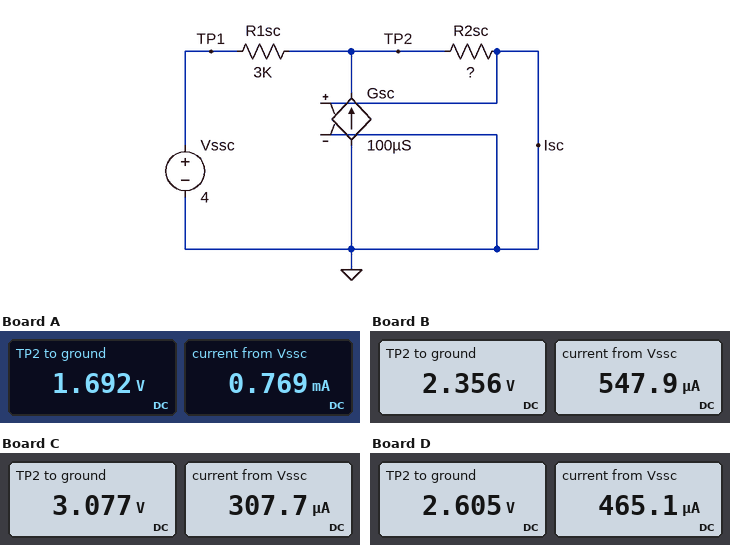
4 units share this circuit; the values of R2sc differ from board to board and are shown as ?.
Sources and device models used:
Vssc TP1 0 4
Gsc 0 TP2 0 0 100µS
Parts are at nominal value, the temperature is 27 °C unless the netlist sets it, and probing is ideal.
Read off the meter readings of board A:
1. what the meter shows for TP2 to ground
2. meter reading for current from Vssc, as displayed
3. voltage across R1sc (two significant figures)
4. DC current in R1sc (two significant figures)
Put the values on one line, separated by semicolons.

1.692 V; 0.769 mA; 2.3 V; 770 µA
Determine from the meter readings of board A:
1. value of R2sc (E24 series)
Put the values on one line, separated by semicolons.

2.2 kΩ
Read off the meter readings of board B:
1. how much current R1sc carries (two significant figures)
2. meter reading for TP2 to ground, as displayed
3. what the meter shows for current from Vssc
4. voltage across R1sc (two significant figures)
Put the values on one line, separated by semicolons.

550 µA; 2.356 V; 547.9 µA; 1.6 V
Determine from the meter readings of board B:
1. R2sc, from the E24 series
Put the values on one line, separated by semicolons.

4.3 kΩ
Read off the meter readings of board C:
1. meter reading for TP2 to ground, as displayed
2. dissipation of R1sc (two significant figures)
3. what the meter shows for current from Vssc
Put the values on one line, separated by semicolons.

3.077 V; 280 µW; 307.7 µA
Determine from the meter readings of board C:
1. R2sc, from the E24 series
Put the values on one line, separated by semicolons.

10 kΩ
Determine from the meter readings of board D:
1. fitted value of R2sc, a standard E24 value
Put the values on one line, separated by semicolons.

5.6 kΩ
